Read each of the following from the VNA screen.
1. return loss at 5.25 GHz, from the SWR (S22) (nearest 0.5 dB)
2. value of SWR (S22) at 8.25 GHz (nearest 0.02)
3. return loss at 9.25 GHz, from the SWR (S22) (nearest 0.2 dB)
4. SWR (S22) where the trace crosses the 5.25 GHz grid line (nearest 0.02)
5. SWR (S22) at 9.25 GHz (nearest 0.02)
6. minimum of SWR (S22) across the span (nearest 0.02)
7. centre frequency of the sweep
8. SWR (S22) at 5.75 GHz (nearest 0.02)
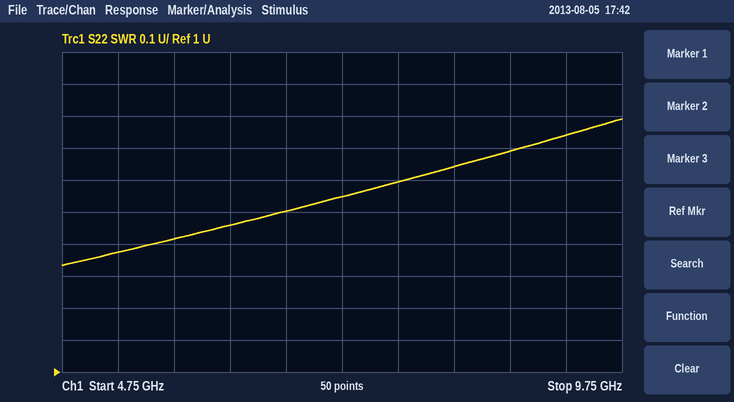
16.0 dB
1.64
11.4 dB
1.38
1.74
1.34
7.25 GHz
1.42
